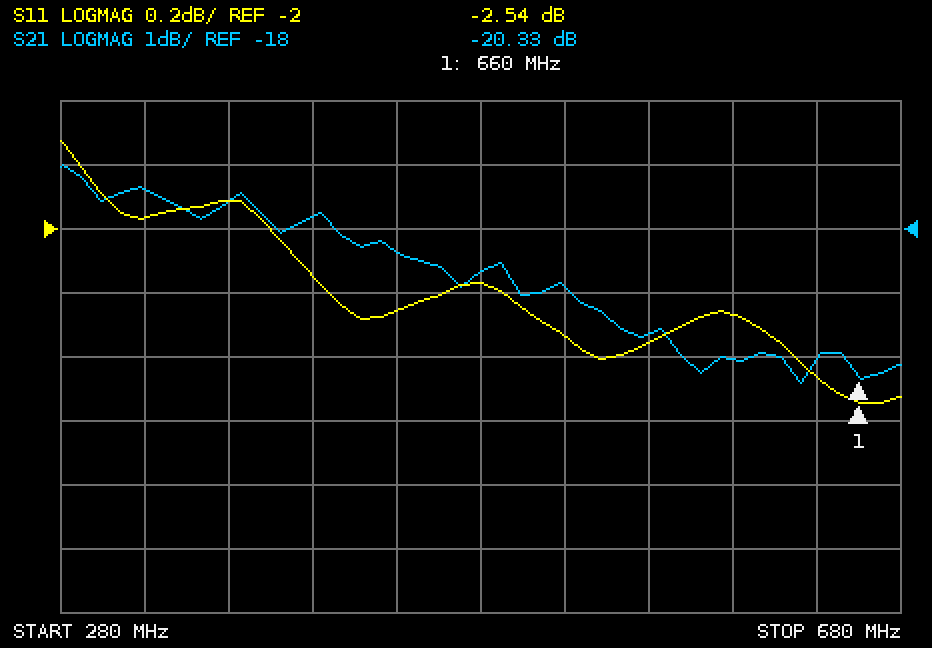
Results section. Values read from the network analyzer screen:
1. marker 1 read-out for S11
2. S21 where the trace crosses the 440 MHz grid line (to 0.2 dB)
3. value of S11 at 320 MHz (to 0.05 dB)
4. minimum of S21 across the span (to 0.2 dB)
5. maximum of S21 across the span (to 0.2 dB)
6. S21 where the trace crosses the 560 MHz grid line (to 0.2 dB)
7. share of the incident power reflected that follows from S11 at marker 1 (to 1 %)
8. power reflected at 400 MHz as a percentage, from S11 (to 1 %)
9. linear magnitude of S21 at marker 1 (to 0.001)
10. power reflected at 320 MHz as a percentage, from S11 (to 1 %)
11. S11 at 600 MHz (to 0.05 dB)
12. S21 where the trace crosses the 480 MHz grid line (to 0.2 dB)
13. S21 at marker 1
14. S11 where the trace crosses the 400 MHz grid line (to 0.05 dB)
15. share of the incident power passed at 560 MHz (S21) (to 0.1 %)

-2.54 dB
-18.4 dB
-1.95 dB
-20.4 dB
-17.0 dB
-19.6 dB
56 %
61 %
0.096
64 %
-2.25 dB
-18.6 dB
-20.33 dB
-2.15 dB
1.1 %
